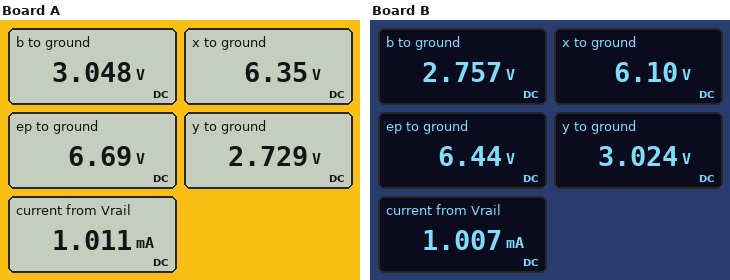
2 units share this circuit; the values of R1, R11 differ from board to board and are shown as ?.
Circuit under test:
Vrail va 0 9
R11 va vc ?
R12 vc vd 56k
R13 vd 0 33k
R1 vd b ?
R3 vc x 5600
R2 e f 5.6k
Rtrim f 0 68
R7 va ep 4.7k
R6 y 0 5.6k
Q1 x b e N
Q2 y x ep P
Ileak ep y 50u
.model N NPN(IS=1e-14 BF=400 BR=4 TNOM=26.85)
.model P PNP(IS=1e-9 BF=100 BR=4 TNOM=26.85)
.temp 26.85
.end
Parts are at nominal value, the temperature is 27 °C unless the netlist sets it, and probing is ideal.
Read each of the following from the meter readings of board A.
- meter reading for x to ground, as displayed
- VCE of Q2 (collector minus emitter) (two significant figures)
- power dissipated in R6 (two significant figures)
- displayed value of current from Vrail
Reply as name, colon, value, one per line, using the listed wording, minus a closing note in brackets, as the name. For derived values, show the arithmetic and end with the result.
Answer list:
meter reading for x to ground, as displayed: 6.35 V
VCE of Q2 (collector minus emitter): 2.729 V - 6.69 V = -4.0 V
power dissipated in R6: (2.729 V)^2 / 5.6 kΩ = 1.3 mW
displayed value of current from Vrail: 1.011 mA
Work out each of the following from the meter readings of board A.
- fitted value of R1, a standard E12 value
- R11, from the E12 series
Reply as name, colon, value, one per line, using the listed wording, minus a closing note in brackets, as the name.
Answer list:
fitted value of R1, a standard E12 value: 150 kΩ
R11, from the E12 series: 560 Ω
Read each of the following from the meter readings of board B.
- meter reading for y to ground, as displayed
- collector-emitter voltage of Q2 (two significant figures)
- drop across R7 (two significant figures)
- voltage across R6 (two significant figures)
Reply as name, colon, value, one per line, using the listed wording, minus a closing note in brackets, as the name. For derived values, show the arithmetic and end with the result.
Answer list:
meter reading for y to ground, as displayed: 3.024 V
collector-emitter voltage of Q2: 3.024 V - 6.44 V = -3.4 V
drop across R7: 9 V - 6.44 V = 2.6 V
voltage across R6: 3.024 V = 3.0 V
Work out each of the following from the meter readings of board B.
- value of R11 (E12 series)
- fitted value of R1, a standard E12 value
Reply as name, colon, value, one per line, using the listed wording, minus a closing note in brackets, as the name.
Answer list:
value of R11: 1.8 kΩ
fitted value of R1, a standard E12 value: 270 kΩ
